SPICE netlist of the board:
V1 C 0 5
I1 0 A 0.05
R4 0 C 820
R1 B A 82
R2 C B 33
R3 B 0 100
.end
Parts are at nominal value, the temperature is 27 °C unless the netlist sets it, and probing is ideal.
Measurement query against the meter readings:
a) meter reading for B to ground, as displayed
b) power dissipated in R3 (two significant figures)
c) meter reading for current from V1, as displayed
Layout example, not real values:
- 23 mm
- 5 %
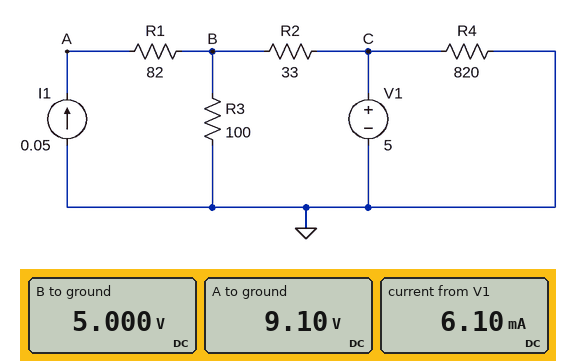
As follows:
- 5.000 V
- 250 mW
- 6.10 mA
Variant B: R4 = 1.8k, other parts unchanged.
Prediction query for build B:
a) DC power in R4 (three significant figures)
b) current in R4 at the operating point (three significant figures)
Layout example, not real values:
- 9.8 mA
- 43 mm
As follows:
- 13.9 mW
- 2.78 mA
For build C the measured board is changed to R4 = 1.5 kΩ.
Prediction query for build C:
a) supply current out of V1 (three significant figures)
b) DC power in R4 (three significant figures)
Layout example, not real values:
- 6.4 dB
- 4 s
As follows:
- 3.33 mA
- 16.7 mW
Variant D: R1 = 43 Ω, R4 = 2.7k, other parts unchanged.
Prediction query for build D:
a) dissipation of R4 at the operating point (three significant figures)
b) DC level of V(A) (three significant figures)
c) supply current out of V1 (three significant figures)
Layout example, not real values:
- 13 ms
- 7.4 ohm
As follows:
- 9.26 mW
- 7.15 V
- 1.85 mA
